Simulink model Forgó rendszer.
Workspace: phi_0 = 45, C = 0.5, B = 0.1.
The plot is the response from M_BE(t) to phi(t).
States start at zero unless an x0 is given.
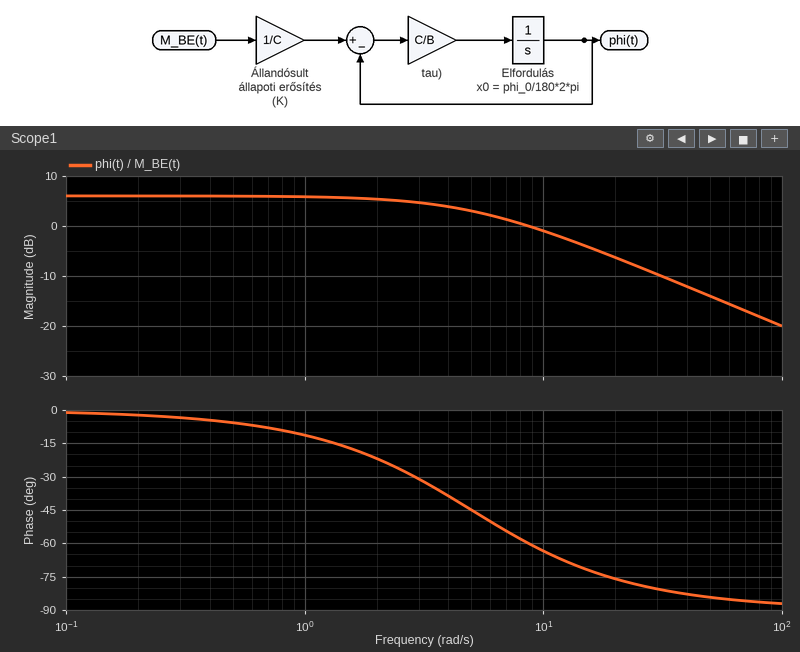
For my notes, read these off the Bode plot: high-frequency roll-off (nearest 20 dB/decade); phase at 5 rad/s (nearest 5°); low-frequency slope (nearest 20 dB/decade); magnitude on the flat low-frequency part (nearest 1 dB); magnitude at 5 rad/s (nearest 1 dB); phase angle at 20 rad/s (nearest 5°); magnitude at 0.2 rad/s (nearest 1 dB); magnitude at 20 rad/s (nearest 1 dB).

-20 dB/decade
-45°
0 dB/decade
6 dB
3 dB
-75°
6 dB
-6 dB
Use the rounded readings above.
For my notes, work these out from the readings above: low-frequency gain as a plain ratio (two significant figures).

2.0
